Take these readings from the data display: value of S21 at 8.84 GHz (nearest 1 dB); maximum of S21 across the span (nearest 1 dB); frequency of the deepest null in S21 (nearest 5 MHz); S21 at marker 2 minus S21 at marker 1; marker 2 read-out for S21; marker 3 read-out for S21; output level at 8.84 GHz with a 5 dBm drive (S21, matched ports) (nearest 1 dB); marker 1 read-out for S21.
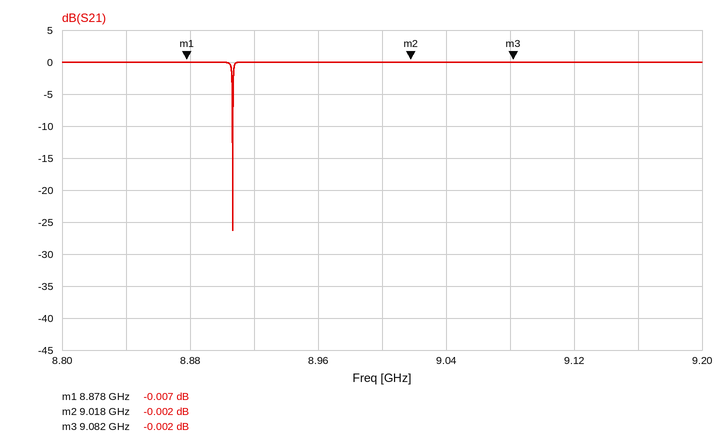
0 dB
0 dB
8.905 GHz
0.005 dB
-0.002 dB
-0.002 dB
5 dBm
-0.007 dB
